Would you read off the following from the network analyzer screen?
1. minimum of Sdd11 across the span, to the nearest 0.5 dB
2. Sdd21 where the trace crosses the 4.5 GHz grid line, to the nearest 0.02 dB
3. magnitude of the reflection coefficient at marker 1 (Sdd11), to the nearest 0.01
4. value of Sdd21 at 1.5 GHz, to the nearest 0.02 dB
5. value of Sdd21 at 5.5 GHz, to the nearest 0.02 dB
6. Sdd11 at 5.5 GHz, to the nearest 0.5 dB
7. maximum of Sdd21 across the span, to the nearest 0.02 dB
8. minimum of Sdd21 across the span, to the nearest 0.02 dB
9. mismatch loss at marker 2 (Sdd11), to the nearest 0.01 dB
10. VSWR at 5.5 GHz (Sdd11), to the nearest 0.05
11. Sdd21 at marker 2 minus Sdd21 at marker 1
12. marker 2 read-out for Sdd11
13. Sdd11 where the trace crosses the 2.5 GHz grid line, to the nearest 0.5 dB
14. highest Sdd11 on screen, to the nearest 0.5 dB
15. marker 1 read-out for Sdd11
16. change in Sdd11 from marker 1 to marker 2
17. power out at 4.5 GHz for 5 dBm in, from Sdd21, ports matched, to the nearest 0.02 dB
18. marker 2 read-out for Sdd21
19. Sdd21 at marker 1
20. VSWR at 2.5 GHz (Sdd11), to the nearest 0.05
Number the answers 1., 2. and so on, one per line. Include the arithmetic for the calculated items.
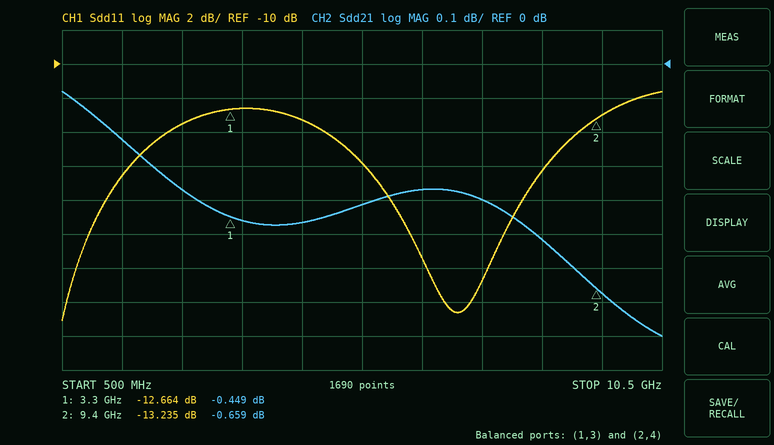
1. -25.0 dB
2. -0.46 dB
3. 10^(-12.664/20) ≈ 0.23
4. -0.22 dB
5. -0.42 dB
6. -16.0 dB
7. -0.08 dB
8. -0.80 dB
9. −10 log10(1 − 10^(-13.235/10)) ≈ 0.21 dB
10. |Γ| = 10^(-16/20) = 0.1585; VSWR = (1 + 0.1585)/(1 − 0.1585) ≈ 1.38, so 1.40 to the nearest 0.05
11. -0.659 − (-0.449) = -0.210 dB
12. -13.235 dB
13. -13.5 dB
14. -11.5 dB
15. -12.664 dB
16. -13.235 − (-12.664) = -0.571 dB
17. 5 dBm + (-0.46 dB) = 4.54 dBm
18. -0.659 dB
19. -0.449 dB
20. |Γ| = 10^(-13.5/20) = 0.2113; VSWR = (1 + 0.2113)/(1 − 0.2113) ≈ 1.54, so 1.55 to the nearest 0.05
